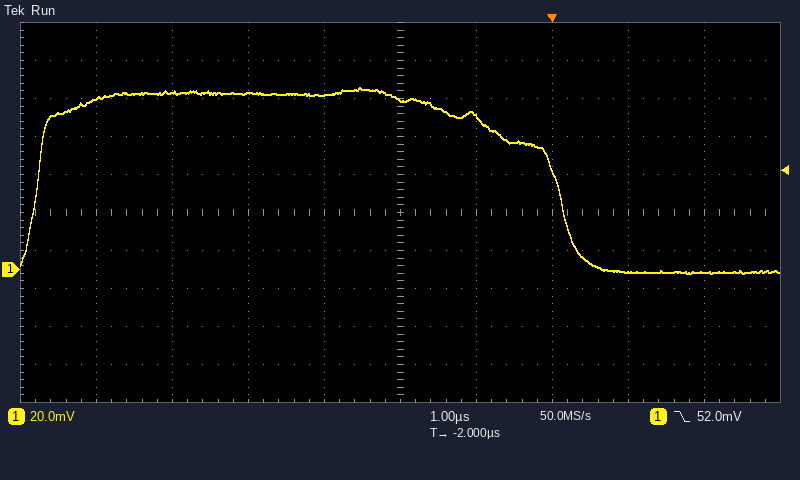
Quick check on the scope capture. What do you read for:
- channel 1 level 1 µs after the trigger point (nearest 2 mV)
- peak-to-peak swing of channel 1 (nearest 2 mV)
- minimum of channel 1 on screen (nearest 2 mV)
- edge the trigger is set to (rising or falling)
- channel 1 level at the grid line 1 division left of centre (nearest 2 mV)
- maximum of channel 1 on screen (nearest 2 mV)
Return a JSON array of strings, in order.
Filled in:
["-2 mV", "98 mV", "-2 mV", "falling", "92 mV", "96 mV"]
